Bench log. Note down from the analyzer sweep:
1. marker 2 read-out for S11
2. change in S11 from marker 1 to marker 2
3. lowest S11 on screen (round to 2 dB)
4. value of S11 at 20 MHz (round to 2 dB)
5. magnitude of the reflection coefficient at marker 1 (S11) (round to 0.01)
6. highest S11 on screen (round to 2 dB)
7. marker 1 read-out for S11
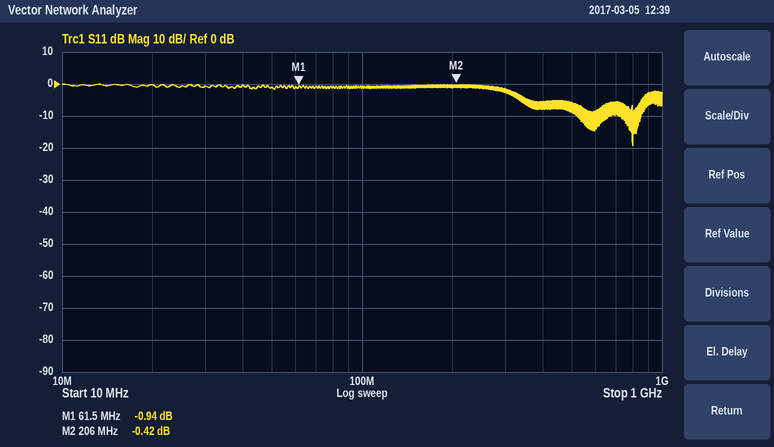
-0.42 dB
0.52 dB
-20 dB
0 dB
0.90
0 dB
-0.94 dB
